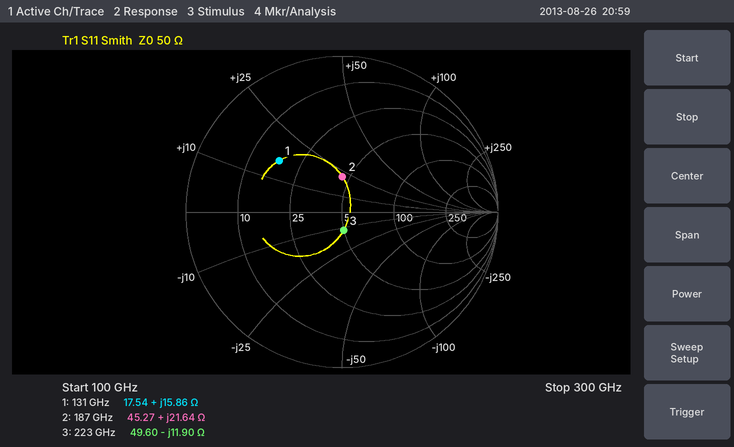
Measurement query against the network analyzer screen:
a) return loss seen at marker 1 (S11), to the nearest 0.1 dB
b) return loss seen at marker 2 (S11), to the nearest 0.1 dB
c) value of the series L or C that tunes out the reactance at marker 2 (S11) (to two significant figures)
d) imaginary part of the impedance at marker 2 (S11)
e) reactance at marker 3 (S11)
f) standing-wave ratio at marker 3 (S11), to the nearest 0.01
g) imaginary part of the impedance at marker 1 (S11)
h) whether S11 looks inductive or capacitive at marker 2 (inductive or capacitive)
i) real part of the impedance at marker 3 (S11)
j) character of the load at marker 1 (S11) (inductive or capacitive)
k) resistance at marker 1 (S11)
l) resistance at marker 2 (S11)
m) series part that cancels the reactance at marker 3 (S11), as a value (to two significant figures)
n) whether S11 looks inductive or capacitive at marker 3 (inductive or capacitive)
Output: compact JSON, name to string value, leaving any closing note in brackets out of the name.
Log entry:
{"return loss seen at marker 1 (S11), to the nearest 0.1 dB": "5.7 dB", "return loss seen at marker 2 (S11), to the nearest 0.1 dB": "12.9 dB", "value of the series L or C that tunes out the reactance at marker 2 (S11)": "39 fF", "imaginary part of the impedance at marker 2": "+21.64 Ω", "reactance at marker 3": "-11.90 Ω", "standing-wave ratio at marker 3 (S11), to the nearest 0.01": "1.27", "imaginary part of the impedance at marker 1": "+15.86 Ω", "whether S11 looks inductive or capacitive at marker 2": "inductive", "real part of the impedance at marker 3": "49.60 Ω", "character of the load at marker 1 (S11)": "inductive", "resistance at marker 1": "17.54 Ω", "resistance at marker 2": "45.27 Ω", "series part that cancels the reactance at marker 3 (S11), as a value": "8.5 pH", "whether S11 looks inductive or capacitive at marker 3": "capacitive"}
